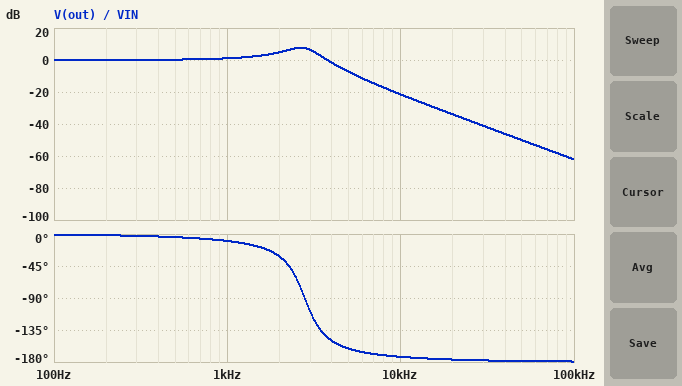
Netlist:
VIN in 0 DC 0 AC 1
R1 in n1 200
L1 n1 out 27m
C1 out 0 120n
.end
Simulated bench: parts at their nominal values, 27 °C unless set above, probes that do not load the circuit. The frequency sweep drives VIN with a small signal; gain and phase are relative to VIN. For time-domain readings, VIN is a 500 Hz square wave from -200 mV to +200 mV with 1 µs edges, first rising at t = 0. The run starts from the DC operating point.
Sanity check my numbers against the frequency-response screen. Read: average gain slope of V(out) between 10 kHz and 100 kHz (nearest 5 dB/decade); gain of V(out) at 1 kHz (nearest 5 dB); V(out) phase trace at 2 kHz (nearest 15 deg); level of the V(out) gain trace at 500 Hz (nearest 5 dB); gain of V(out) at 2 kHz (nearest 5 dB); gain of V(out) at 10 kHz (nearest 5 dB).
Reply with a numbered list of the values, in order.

1. -40 dB/decade
2. 0 dB
3. -30 deg
4. 0 dB
5. 5 dB
6. -20 dB
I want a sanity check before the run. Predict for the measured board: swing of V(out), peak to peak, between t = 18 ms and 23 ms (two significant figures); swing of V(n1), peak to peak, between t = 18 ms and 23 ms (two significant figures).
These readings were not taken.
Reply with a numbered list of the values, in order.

1. 810 mV
2. 530 mV
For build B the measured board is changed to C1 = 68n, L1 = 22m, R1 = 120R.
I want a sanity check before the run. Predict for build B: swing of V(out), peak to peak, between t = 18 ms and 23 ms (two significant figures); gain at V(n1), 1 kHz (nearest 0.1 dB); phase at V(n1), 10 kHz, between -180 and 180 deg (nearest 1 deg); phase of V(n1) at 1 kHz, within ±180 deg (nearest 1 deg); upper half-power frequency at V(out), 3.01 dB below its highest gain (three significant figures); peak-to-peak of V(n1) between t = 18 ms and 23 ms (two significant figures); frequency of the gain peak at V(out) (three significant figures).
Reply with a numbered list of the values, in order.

1. 940 mV
2. 0 dB
3. 6 deg
4. -3 deg
5. 4.48 kHz
6. 500 mV
7. 4.07 kHz
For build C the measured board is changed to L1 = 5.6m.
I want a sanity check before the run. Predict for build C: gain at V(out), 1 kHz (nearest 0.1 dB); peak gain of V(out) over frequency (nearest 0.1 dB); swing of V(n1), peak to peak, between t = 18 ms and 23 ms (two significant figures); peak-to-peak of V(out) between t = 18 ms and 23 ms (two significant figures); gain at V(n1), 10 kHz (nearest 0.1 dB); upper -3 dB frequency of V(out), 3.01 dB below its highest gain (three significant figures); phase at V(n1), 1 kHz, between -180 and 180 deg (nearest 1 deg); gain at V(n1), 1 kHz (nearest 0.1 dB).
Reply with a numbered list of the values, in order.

1. 0.1 dB
2. 1.7 dB
3. 480 mV
4. 560 mV
5. -2.6 dB
6. 7.24 kHz
7. -9 deg
8. -0.1 dB
